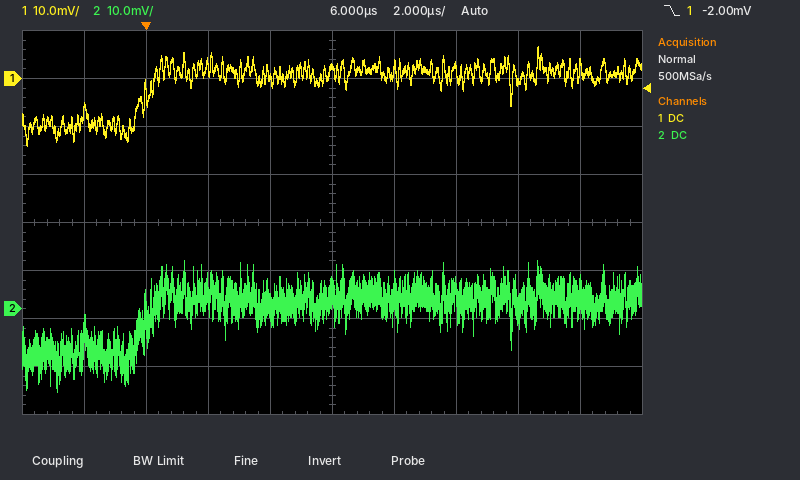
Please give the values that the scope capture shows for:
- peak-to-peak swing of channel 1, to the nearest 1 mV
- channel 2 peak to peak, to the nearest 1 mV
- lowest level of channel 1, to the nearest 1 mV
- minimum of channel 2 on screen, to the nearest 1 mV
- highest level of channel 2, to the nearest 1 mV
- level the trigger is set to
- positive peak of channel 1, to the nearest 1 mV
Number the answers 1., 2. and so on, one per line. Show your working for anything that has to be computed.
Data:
1. 7 mV − (-14 mV) = 21 mV
2. 10 mV − (-17 mV) = 27 mV
3. -14 mV
4. -17 mV
5. 10 mV
6. -2.00 mV
7. 7 mV
